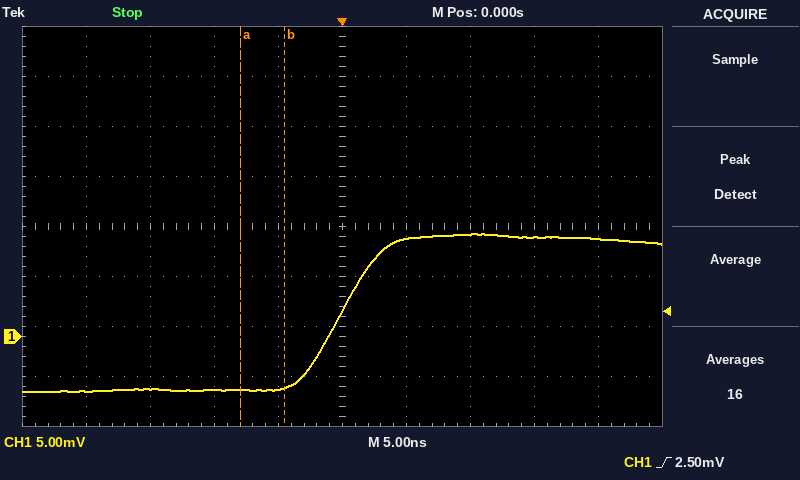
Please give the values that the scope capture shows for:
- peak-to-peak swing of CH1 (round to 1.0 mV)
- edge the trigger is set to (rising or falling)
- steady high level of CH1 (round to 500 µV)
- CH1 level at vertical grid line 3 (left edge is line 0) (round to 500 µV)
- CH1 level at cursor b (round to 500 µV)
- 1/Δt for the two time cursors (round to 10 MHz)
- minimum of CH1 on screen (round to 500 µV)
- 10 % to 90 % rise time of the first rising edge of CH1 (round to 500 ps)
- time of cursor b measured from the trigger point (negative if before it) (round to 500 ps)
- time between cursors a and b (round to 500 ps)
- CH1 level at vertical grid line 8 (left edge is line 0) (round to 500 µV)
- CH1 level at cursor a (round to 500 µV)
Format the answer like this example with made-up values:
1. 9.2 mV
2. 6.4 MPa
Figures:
1. 16.0 mV
2. rising
3. 10.0 mV
4. -5.5 mV
5. -5.0 mV
6. 290 MHz
7. -5.5 mV
8. 6.0 ns
9. -4.5 ns
10. 3.5 ns
11. 10.0 mV
12. -5.5 mV
